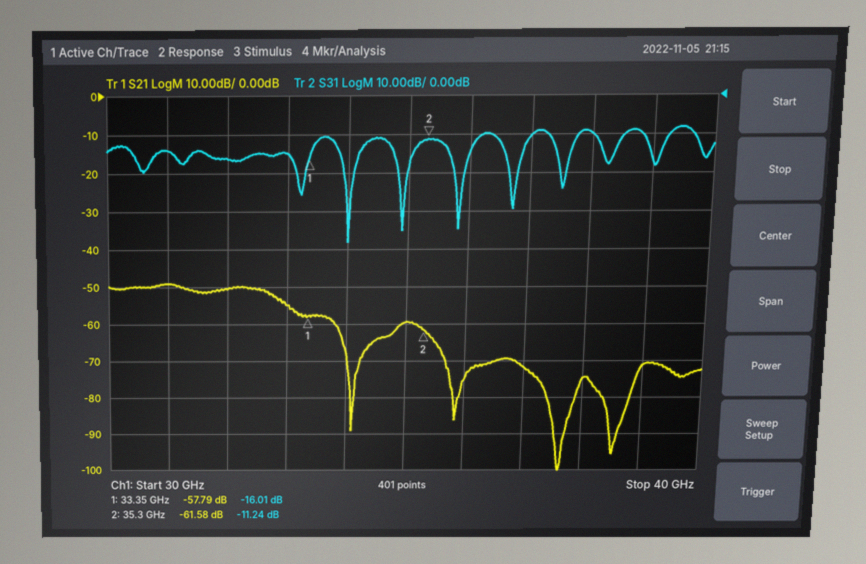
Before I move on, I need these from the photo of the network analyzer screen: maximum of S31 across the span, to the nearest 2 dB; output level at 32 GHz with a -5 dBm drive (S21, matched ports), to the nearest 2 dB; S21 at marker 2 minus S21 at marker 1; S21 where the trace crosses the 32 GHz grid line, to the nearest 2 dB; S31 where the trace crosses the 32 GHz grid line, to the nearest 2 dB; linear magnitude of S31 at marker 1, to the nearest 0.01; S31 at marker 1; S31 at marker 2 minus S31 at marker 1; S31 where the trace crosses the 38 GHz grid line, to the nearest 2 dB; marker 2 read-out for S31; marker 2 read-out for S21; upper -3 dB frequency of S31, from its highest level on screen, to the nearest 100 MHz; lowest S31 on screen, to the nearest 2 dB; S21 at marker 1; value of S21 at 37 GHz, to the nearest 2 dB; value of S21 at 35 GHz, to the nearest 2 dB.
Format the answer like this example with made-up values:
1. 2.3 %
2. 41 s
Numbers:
1. -8 dB
2. -56 dBm
3. -3.79 dB
4. -50 dB
5. -16 dB
6. 0.16
7. -16.01 dB
8. 4.77 dB
9. -10 dB
10. -11.24 dB
11. -61.58 dB
12. 39.7 GHz
13. -38 dB
14. -57.79 dB
15. -72 dB
16. -60 dB
